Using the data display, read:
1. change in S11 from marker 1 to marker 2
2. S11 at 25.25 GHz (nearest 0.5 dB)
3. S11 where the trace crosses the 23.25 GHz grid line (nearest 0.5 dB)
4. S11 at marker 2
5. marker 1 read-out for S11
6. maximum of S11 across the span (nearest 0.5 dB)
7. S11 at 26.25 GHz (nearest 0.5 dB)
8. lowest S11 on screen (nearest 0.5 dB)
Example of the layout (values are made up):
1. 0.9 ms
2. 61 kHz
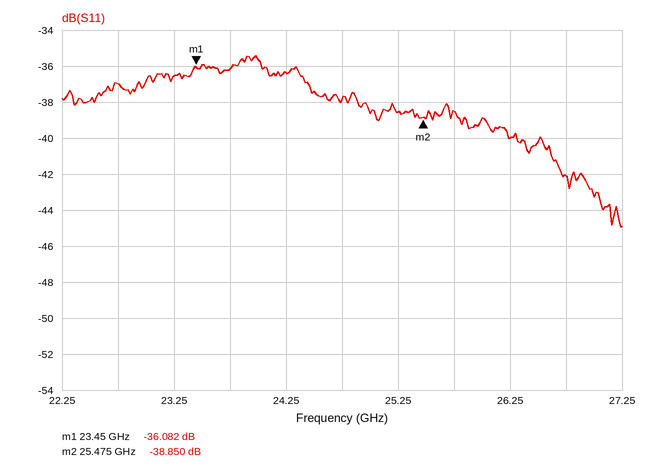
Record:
1. -2.768 dB
2. -38.5 dB
3. -36.5 dB
4. -38.850 dB
5. -36.082 dB
6. -35.5 dB
7. -40.0 dB
8. -45.0 dB
